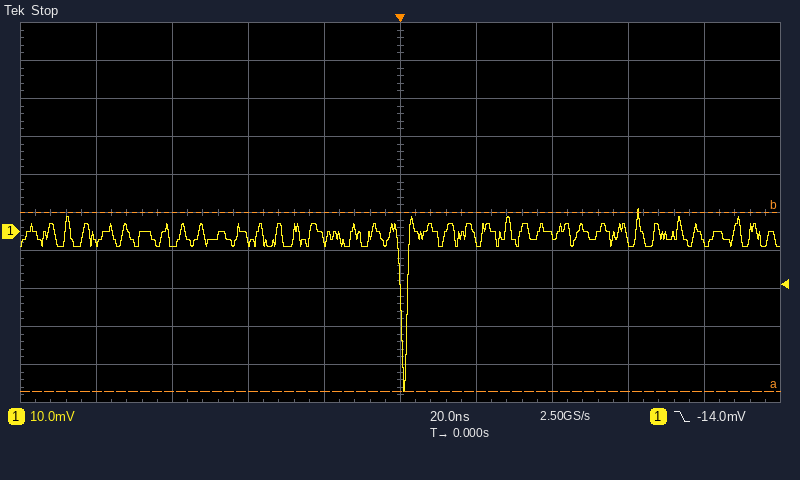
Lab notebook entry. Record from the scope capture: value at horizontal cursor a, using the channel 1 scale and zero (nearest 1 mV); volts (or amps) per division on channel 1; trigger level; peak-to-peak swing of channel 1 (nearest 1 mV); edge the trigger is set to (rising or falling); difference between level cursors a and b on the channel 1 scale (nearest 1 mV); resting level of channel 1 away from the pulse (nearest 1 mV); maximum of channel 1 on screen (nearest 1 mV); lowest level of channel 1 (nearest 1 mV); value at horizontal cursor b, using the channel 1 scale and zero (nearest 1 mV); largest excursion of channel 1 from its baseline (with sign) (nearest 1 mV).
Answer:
-42 mV
10 mV
-14.0 mV
48 mV
falling
47 mV
-1 mV
6 mV
-42 mV
5 mV
-41 mV
